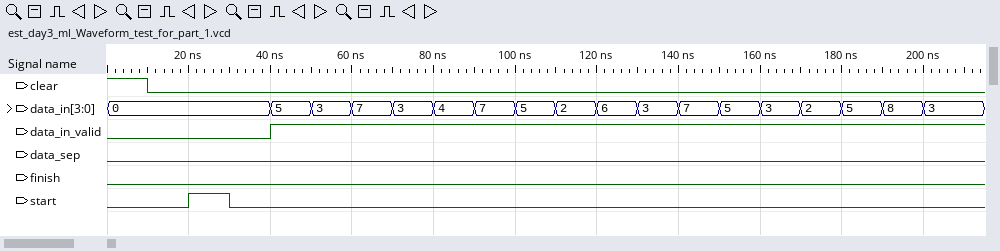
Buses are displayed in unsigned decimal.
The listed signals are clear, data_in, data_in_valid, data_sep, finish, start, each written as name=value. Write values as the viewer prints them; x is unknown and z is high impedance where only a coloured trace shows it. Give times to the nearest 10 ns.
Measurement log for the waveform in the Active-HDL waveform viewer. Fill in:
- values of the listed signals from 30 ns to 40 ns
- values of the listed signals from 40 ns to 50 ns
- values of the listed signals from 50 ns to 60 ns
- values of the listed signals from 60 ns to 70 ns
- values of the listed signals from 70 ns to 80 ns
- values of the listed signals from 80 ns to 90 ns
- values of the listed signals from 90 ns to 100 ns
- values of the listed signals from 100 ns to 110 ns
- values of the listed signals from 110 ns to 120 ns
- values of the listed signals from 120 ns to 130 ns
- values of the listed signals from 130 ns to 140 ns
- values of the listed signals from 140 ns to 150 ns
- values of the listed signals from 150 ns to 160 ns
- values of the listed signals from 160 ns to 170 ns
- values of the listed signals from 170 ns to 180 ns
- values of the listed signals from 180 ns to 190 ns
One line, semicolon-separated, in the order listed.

clear=0, data_in=0, data_in_valid=0, data_sep=0, finish=0, start=0; clear=0, data_in=5, data_in_valid=1, data_sep=0, finish=0, start=0; clear=0, data_in=3, data_in_valid=1, data_sep=0, finish=0, start=0; clear=0, data_in=7, data_in_valid=1, data_sep=0, finish=0, start=0; clear=0, data_in=3, data_in_valid=1, data_sep=0, finish=0, start=0; clear=0, data_in=4, data_in_valid=1, data_sep=0, finish=0, start=0; clear=0, data_in=7, data_in_valid=1, data_sep=0, finish=0, start=0; clear=0, data_in=5, data_in_valid=1, data_sep=0, finish=0, start=0; clear=0, data_in=2, data_in_valid=1, data_sep=0, finish=0, start=0; clear=0, data_in=6, data_in_valid=1, data_sep=0, finish=0, start=0; clear=0, data_in=3, data_in_valid=1, data_sep=0, finish=0, start=0; clear=0, data_in=7, data_in_valid=1, data_sep=0, finish=0, start=0; clear=0, data_in=5, data_in_valid=1, data_sep=0, finish=0, start=0; clear=0, data_in=3, data_in_valid=1, data_sep=0, finish=0, start=0; clear=0, data_in=2, data_in_valid=1, data_sep=0, finish=0, start=0; clear=0, data_in=5, data_in_valid=1, data_sep=0, finish=0, start=0
